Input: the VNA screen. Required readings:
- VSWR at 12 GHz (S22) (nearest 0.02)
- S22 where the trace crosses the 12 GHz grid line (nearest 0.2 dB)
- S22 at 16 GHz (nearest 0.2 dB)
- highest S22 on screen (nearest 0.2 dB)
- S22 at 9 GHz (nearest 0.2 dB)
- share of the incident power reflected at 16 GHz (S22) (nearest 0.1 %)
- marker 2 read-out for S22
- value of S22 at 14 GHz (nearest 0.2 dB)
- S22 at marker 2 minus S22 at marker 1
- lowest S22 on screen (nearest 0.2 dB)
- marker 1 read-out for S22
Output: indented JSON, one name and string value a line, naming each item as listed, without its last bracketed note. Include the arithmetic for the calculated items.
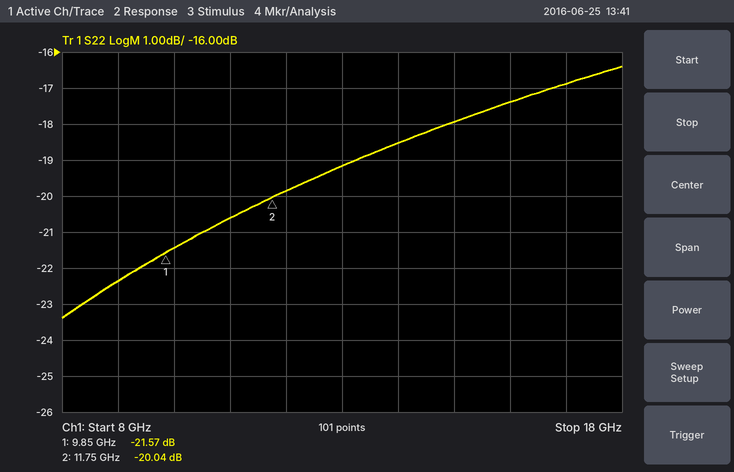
{
  "VSWR at 12 GHz (S22)": "|Γ| = 10^(-19.8/20) = 0.1023; VSWR = (1 + 0.1023)/(1 − 0.1023) ≈ 1.23, so 1.22 to the nearest 0.02",
  "S22 where the trace crosses the 12 GHz grid line": "-19.8 dB",
  "S22 at 16 GHz": "-17.4 dB",
  "highest S22 on screen": "-16.4 dB",
  "S22 at 9 GHz": "-22.4 dB",
  "share of the incident power reflected at 16 GHz (S22)": "10^(-17.4/10) ≈ 1.8 %",
  "marker 2 read-out for S22": "-20.04 dB",
  "value of S22 at 14 GHz": "-18.6 dB",
  "S22 at marker 2 minus S22 at marker 1": "-20.04 − (-21.57) = 1.53 dB",
  "lowest S22 on screen": "-23.4 dB",
  "marker 1 read-out for S22": "-21.57 dB"
}
